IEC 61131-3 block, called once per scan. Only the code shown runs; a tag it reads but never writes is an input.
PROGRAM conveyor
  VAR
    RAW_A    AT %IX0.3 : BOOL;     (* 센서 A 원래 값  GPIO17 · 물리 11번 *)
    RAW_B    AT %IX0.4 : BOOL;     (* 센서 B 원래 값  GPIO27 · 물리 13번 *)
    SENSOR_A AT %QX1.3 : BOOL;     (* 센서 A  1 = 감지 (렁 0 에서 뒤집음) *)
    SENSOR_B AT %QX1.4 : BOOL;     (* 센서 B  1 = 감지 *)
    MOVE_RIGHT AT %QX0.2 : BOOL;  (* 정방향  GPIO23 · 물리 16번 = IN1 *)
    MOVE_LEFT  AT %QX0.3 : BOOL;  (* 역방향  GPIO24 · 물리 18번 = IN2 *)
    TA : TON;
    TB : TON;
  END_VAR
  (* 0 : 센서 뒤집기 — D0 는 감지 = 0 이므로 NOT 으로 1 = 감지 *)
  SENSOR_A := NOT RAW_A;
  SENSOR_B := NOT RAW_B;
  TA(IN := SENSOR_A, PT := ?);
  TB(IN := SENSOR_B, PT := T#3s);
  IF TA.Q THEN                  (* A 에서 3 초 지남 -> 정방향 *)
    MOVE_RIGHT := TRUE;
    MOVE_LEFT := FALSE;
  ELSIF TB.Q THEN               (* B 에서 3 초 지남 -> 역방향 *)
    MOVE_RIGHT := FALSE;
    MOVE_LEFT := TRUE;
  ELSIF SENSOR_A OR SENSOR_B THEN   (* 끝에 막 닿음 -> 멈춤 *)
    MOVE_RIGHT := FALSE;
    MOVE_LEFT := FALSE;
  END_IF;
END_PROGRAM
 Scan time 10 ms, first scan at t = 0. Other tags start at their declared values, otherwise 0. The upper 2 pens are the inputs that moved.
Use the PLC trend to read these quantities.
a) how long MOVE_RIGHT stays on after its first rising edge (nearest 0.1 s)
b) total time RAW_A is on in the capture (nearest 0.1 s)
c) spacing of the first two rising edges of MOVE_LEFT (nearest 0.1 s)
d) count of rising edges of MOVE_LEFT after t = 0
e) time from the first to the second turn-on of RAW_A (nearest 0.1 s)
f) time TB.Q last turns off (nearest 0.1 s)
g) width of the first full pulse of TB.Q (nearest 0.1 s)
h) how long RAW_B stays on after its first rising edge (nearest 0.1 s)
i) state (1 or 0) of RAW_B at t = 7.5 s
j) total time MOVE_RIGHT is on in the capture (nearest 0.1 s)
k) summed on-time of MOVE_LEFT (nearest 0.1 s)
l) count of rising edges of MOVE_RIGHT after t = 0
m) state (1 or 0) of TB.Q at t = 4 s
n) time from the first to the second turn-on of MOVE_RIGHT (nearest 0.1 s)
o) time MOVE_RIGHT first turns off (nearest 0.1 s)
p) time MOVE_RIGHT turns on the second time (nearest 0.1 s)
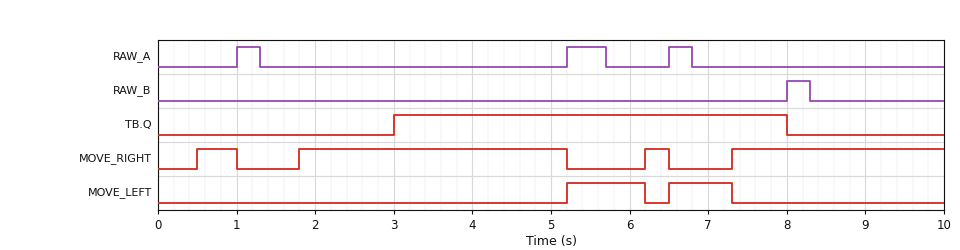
0.5 s
1.1 s
1.3 s
2
4.2 s
8.0 s
5.0 s
0.3 s
0
6.9 s
1.8 s
4
1
1.3 s
1.0 s
1.8 s
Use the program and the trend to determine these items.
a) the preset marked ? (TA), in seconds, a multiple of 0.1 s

0.5 s
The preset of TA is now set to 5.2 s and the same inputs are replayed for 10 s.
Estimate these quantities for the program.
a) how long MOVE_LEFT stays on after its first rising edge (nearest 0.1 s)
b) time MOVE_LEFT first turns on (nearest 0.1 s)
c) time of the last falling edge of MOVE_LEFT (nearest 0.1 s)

5.0 s
3.0 s
8.0 s
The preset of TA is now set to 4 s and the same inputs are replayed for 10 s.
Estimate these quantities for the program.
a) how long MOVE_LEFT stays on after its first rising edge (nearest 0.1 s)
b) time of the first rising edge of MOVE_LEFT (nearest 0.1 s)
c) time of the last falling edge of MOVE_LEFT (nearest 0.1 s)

5.0 s
3.0 s
8.0 s
